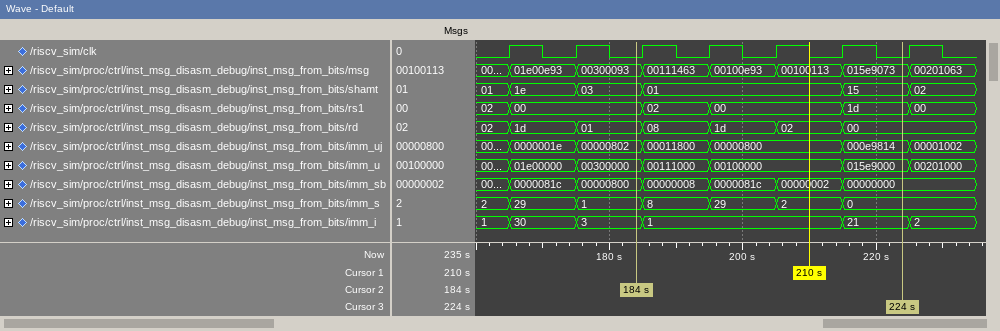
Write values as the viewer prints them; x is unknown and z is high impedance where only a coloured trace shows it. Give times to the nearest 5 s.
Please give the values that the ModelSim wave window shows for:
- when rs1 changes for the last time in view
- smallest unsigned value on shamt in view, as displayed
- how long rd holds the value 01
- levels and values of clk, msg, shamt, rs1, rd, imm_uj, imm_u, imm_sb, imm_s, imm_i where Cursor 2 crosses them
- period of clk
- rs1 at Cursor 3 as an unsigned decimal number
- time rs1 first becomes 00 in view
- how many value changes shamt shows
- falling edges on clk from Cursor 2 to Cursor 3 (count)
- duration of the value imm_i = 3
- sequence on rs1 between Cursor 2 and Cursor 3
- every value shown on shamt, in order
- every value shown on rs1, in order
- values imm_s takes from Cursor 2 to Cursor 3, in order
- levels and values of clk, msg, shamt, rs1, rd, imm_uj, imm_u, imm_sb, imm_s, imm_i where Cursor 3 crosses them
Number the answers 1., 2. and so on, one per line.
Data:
1. 225 s
2. 01
3. 10 s
4. clk=0, msg=00300093, shamt=03, rs1=00, rd=01, imm_uj=00000802, imm_u=00300000, imm_sb=00000800, imm_s=1, imm_i=3
5. 10 s
6. 29
7. 165 s
8. 5
9. 4
10. 10 s
11. 00, 02, 00, 1d
12. 01, 1e, 03, 01, 15, 02
13. 02, 00, 02, 00, 1d, 00
14. 1, 8, 29, 2, 0
15. clk=0, msg=015e9073, shamt=15, rs1=1d, rd=00, imm_uj=000e9814, imm_u=015e9000, imm_sb=00000000, imm_s=0, imm_i=21
